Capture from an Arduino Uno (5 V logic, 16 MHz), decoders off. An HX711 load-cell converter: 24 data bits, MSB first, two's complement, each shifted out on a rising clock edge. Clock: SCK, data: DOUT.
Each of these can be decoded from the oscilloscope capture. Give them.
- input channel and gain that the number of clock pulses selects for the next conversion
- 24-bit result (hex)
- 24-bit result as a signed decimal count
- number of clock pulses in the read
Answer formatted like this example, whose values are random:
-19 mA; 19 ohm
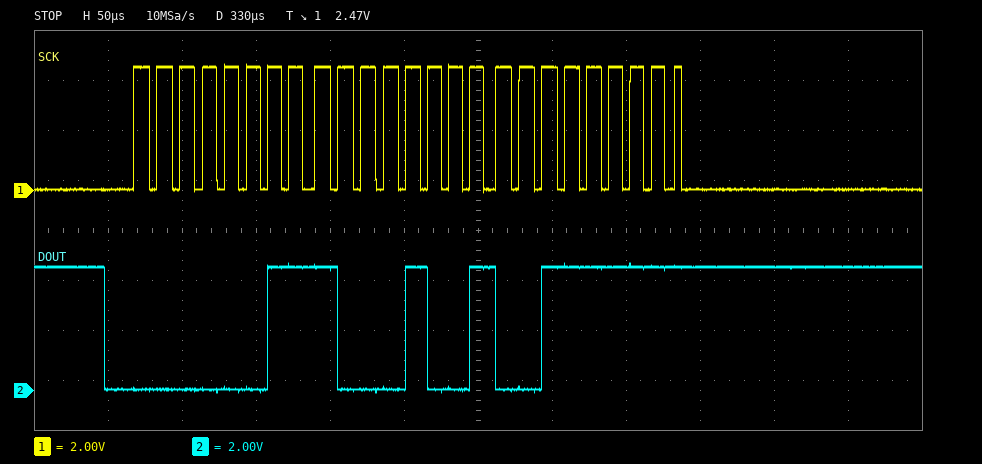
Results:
channel A, gain 128; 0x03893F; 231743; 25
